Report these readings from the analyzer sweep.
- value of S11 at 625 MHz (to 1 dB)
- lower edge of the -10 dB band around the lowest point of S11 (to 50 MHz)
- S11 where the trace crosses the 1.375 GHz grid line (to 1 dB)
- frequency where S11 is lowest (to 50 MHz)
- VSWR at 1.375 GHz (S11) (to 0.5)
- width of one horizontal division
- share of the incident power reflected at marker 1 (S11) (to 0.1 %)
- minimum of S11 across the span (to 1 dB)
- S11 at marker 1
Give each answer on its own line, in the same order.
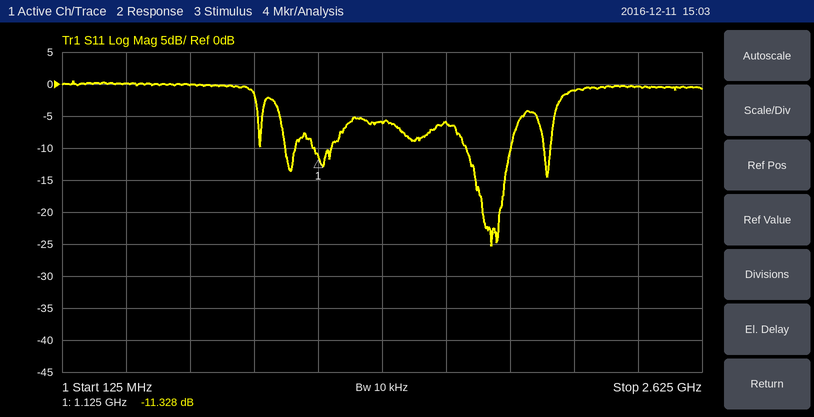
0 dB
1.70 GHz
-6 dB
1.80 GHz
3.0
250 MHz
7.4 %
-25 dB
-11.328 dB
